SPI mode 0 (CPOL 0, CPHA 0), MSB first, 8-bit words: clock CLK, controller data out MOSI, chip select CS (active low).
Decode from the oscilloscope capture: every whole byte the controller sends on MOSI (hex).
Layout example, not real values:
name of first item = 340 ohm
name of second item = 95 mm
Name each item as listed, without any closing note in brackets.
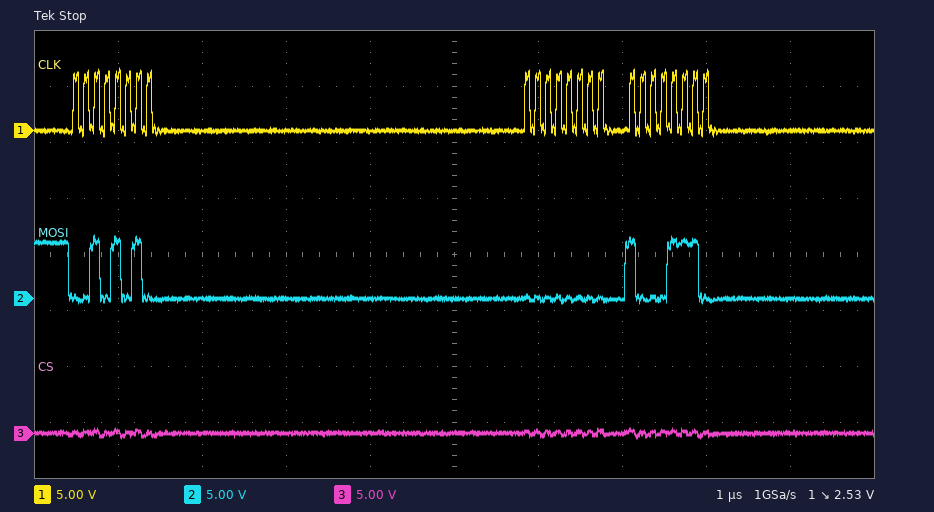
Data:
every whole byte the controller sends on MOSI = 2A 00 8E
